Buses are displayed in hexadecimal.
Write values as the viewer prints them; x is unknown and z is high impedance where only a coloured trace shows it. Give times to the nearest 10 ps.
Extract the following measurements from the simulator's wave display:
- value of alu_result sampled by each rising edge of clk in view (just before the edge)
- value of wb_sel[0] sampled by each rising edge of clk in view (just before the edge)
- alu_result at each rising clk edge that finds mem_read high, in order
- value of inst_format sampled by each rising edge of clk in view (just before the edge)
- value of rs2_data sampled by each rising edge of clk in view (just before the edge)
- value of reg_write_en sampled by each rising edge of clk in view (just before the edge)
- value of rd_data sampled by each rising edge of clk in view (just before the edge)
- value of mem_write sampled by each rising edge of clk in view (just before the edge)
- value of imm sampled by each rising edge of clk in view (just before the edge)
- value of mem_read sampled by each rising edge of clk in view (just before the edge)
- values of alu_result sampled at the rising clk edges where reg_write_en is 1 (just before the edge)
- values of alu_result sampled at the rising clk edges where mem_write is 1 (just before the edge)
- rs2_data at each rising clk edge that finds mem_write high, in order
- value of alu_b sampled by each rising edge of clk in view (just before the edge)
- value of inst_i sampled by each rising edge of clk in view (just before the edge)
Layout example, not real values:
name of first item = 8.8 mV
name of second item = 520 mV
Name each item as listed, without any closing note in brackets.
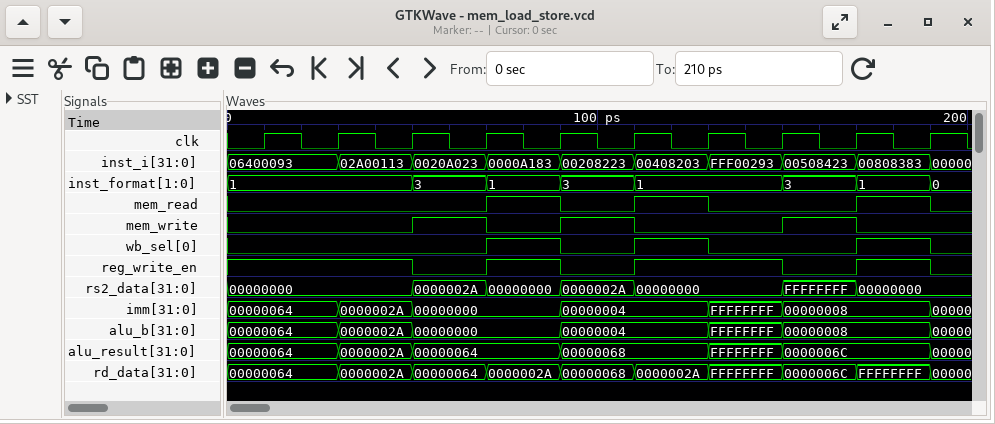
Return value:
value of alu_result sampled by each rising edge of clk in view = 00000064, 00000064, 0000002A, 00000064, 00000064, 00000068, 00000068, FFFFFFFF, 0000006C, 0000006C
value of wb_sel[0] sampled by each rising edge of clk in view = 0 0 0 0 1 0 1 0 0 1
alu_result at each rising clk edge that finds mem_read high, in order = 00000064, 00000068, 0000006C
value of inst_format sampled by each rising edge of clk in view = 1, 1, 1, 3, 1, 3, 1, 1, 3, 1
value of rs2_data sampled by each rising edge of clk in view = 00000000, 00000000, 00000000, 0000002A, 00000000, 0000002A, 00000000, 00000000, FFFFFFFF, 00000000
value of reg_write_en sampled by each rising edge of clk in view = 1 1 1 0 1 0 1 1 0 1
value of rd_data sampled by each rising edge of clk in view = 00000064, 00000064, 0000002A, 00000064, 0000002A, 00000068, 0000002A, FFFFFFFF, 0000006C, FFFFFFFF
value of mem_write sampled by each rising edge of clk in view = 0 0 0 1 0 1 0 0 1 0
value of imm sampled by each rising edge of clk in view = 00000064, 00000064, 0000002A, 00000000, 00000000, 00000004, 00000004, FFFFFFFF, 00000008, 00000008
value of mem_read sampled by each rising edge of clk in view = 0 0 0 0 1 0 1 0 0 1
values of alu_result sampled at the rising clk edges where reg_write_en is 1 = 00000064, 00000064, 0000002A, 00000064, 00000068, FFFFFFFF, 0000006C
values of alu_result sampled at the rising clk edges where mem_write is 1 = 00000064, 00000068, 0000006C
rs2_data at each rising clk edge that finds mem_write high, in order = 0000002A, 0000002A, FFFFFFFF
value of alu_b sampled by each rising edge of clk in view = 00000064, 00000064, 0000002A, 00000000, 00000000, 00000004, 00000004, FFFFFFFF, 00000008, 00000008
value of inst_i sampled by each rising edge of clk in view = 06400093, 06400093, 02A00113, 0020A023, 0000A183, 00208223, 00408203, FFF00293, 00508423, 00808383
